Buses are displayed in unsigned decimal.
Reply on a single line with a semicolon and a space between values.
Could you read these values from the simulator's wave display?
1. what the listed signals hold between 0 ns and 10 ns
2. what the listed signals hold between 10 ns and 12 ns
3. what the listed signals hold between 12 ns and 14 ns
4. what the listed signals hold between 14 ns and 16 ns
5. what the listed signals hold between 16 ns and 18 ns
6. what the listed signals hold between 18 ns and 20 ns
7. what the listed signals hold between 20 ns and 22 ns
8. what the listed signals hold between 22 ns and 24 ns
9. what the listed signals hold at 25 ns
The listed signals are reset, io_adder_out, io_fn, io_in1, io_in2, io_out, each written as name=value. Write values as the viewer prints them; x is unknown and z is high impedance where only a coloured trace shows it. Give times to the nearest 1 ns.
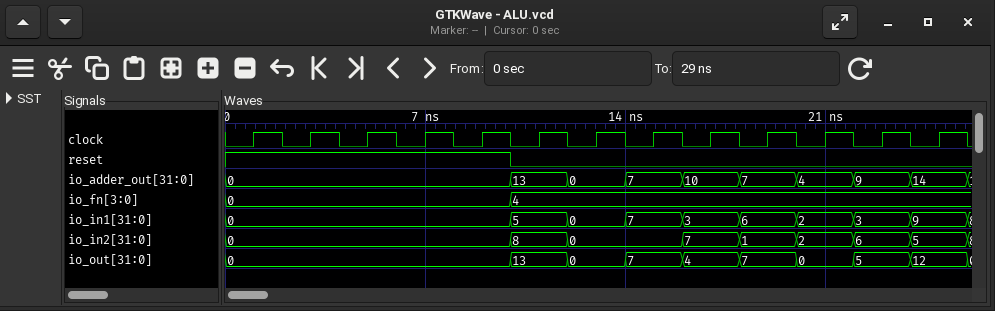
reset=1, io_adder_out=0, io_fn=0, io_in1=0, io_in2=0, io_out=0; reset=0, io_adder_out=13, io_fn=4, io_in1=5, io_in2=8, io_out=13; reset=0, io_adder_out=0, io_fn=4, io_in1=0, io_in2=0, io_out=0; reset=0, io_adder_out=7, io_fn=4, io_in1=7, io_in2=0, io_out=7; reset=0, io_adder_out=10, io_fn=4, io_in1=3, io_in2=7, io_out=4; reset=0, io_adder_out=7, io_fn=4, io_in1=6, io_in2=1, io_out=7; reset=0, io_adder_out=4, io_fn=4, io_in1=2, io_in2=2, io_out=0; reset=0, io_adder_out=9, io_fn=4, io_in1=3, io_in2=6, io_out=5; reset=0, io_adder_out=14, io_fn=4, io_in1=9, io_in2=5, io_out=12
